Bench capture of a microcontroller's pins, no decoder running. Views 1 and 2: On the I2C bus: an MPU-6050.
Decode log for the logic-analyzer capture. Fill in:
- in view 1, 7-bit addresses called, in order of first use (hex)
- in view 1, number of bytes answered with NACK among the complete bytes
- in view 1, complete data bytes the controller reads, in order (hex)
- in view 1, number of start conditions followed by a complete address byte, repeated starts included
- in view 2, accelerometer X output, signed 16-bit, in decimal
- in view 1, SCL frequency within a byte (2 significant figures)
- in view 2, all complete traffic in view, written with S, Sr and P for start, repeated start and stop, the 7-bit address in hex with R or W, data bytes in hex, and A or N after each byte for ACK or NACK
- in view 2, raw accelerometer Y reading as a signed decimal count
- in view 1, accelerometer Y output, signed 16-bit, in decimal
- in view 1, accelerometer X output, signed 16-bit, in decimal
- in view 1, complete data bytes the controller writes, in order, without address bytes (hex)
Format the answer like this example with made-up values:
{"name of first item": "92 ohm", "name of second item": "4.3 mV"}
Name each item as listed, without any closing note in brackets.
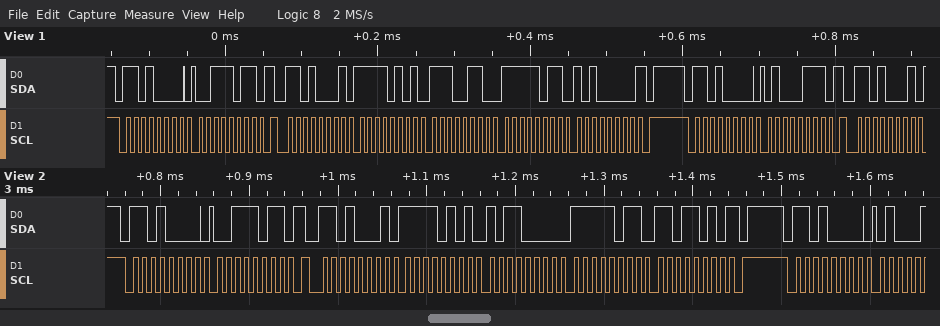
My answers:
{"in view 1, 7-bit addresses called, in order of first use": "0x68", "in view 1, number of bytes answered with NACK among the complete bytes": "1", "in view 1, complete data bytes the controller reads, in order": "F5 E6 FB A0", "in view 1, number of start conditions followed by a complete address byte, repeated starts included": "4", "in view 2, accelerometer X output, signed 16-bit, in decimal": "-2640", "in view 1, SCL frequency within a byte": "100 kHz", "in view 2, all complete traffic in view, written with S, Sr and P for start, repeated start and stop, the 7-bit address in hex with R or W, data bytes in hex, and A or N after each byte for ACK or NACK": "S 68W A 3B A Sr 68R A F5 A B0 A FB A DA N P S 68W A", "in view 2, raw accelerometer Y reading as a signed decimal count": "-1062", "in view 1, accelerometer Y output, signed 16-bit, in decimal": "-1120", "in view 1, accelerometer X output, signed 16-bit, in decimal": "-2586", "in view 1, complete data bytes the controller writes, in order, without address bytes": "3B 47"}
